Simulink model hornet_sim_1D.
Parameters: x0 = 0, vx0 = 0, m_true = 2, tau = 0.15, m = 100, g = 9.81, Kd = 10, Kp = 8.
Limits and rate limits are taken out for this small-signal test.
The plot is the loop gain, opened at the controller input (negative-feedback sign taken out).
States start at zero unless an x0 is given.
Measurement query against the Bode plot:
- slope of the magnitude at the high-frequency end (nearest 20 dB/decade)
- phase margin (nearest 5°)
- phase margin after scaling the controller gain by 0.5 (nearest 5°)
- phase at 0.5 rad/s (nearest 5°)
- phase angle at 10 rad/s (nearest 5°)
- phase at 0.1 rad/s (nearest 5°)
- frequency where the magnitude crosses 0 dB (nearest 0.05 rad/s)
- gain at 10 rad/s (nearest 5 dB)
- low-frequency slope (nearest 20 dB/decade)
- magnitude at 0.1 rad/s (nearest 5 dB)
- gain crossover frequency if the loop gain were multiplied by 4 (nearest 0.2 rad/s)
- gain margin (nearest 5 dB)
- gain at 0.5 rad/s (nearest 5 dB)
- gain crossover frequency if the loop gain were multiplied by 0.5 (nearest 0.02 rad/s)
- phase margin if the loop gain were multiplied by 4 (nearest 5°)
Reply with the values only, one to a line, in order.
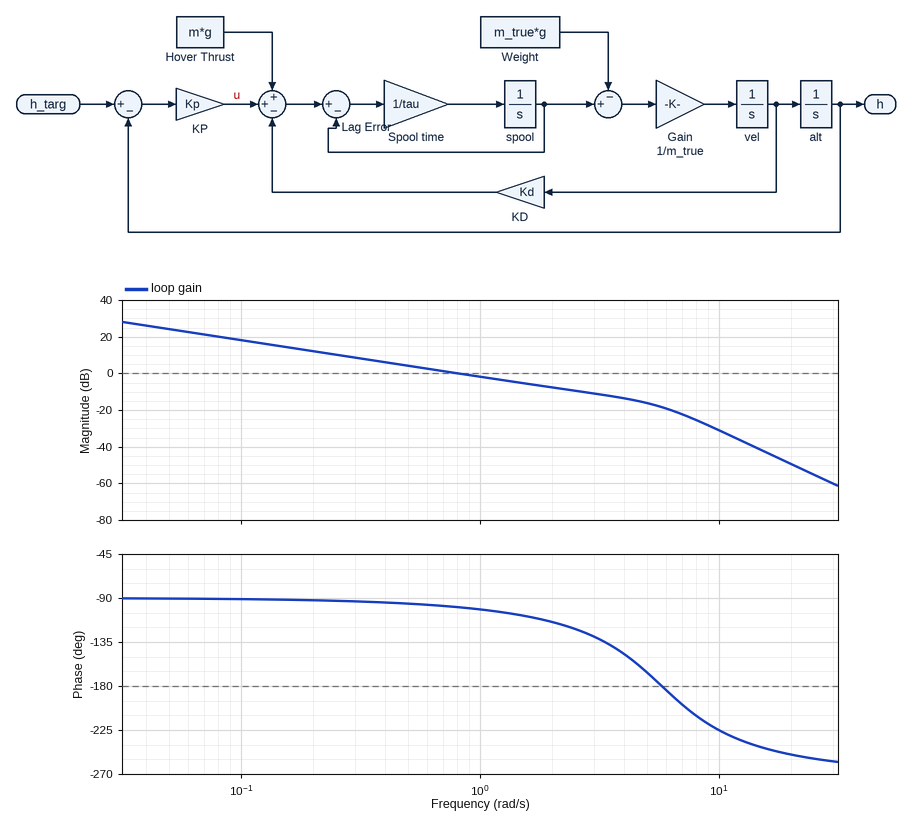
-60 dB/decade
80°
85°
-95°
-225°
-90°
0.80 rad/s
-30 dB
-20 dB/decade
20 dB
3.4 rad/s
20 dB
5 dB
0.40 rad/s
45°
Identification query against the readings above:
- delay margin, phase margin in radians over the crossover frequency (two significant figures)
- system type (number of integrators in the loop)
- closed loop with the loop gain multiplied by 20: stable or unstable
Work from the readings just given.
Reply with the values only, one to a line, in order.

1.7 s
1
unstable
